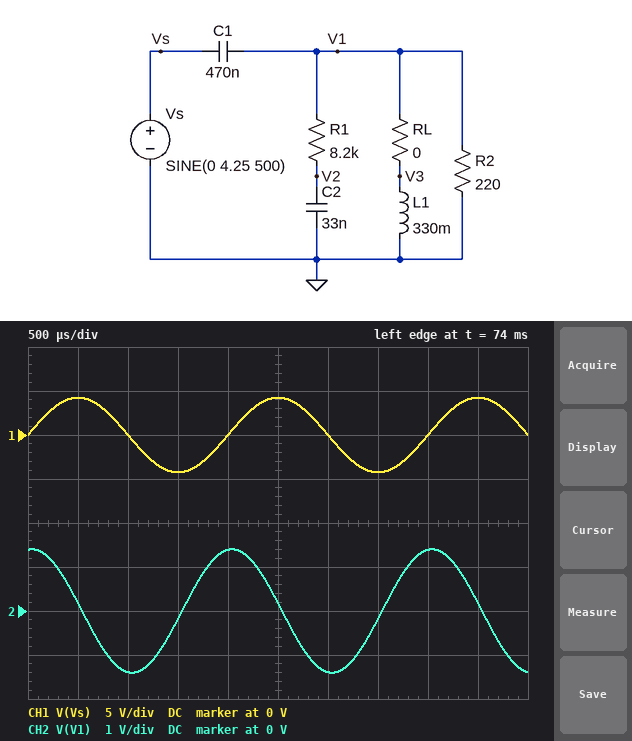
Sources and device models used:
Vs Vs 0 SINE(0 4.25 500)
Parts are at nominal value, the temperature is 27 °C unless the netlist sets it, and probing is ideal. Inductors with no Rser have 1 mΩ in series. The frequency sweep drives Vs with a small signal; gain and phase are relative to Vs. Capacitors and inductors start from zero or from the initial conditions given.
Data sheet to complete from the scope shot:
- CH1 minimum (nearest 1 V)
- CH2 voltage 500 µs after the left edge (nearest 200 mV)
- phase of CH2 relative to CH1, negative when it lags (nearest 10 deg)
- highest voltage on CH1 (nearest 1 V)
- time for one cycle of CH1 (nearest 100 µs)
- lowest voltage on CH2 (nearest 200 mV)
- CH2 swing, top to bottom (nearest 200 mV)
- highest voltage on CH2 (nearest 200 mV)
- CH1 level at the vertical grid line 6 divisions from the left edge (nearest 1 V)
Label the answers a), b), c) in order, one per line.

a) -4 V
b) 200 mV
c) 80 deg
d) 4 V
e) 2.0 ms
f) -1.4 V
g) 2.8 V
h) 1.4 V
i) 0 V
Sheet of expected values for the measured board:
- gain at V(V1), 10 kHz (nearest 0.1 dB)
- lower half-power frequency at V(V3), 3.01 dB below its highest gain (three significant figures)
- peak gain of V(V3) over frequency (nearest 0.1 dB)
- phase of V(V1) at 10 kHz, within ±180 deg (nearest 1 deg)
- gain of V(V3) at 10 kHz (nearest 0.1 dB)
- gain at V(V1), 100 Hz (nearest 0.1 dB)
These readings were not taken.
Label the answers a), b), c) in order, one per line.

a) -0.1 dB
b) 1.48 kHz
c) 0 dB
d) 9 deg
e) -0.1 dB
f) -26.6 dB
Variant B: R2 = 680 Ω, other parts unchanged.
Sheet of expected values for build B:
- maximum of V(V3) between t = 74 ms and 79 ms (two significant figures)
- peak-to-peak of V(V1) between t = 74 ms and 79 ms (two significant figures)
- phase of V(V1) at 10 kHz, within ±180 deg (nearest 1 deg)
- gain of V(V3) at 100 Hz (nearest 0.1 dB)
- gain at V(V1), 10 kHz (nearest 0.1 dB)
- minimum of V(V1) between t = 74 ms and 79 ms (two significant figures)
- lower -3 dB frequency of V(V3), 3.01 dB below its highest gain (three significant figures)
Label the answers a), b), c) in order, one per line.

a) 3.9 V
b) 7.8 V
c) 3 deg
d) -24.1 dB
e) 0 dB
f) -3.9 V
g) 356 Hz
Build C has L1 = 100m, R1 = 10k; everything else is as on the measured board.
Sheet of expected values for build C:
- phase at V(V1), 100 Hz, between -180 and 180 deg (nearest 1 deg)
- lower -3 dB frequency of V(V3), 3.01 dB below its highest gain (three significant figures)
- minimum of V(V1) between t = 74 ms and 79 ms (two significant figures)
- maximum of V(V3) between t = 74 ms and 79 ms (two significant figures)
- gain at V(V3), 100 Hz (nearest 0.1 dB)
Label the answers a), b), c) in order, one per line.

a) 164 deg
b) 1.26 kHz
c) -1.3 V
d) 1.3 V
e) -34.8 dB
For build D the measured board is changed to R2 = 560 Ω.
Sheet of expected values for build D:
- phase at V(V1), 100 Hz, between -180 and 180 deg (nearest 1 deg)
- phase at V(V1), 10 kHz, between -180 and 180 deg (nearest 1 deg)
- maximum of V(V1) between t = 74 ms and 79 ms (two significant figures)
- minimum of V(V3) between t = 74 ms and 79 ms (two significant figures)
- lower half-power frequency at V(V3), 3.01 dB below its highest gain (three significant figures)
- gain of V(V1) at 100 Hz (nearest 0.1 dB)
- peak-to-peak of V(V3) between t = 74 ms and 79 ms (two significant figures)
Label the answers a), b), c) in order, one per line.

a) 158 deg
b) 4 deg
c) 3.2 V
d) -3.2 V
e) 444 Hz
f) -24.3 dB
g) 6.4 V
